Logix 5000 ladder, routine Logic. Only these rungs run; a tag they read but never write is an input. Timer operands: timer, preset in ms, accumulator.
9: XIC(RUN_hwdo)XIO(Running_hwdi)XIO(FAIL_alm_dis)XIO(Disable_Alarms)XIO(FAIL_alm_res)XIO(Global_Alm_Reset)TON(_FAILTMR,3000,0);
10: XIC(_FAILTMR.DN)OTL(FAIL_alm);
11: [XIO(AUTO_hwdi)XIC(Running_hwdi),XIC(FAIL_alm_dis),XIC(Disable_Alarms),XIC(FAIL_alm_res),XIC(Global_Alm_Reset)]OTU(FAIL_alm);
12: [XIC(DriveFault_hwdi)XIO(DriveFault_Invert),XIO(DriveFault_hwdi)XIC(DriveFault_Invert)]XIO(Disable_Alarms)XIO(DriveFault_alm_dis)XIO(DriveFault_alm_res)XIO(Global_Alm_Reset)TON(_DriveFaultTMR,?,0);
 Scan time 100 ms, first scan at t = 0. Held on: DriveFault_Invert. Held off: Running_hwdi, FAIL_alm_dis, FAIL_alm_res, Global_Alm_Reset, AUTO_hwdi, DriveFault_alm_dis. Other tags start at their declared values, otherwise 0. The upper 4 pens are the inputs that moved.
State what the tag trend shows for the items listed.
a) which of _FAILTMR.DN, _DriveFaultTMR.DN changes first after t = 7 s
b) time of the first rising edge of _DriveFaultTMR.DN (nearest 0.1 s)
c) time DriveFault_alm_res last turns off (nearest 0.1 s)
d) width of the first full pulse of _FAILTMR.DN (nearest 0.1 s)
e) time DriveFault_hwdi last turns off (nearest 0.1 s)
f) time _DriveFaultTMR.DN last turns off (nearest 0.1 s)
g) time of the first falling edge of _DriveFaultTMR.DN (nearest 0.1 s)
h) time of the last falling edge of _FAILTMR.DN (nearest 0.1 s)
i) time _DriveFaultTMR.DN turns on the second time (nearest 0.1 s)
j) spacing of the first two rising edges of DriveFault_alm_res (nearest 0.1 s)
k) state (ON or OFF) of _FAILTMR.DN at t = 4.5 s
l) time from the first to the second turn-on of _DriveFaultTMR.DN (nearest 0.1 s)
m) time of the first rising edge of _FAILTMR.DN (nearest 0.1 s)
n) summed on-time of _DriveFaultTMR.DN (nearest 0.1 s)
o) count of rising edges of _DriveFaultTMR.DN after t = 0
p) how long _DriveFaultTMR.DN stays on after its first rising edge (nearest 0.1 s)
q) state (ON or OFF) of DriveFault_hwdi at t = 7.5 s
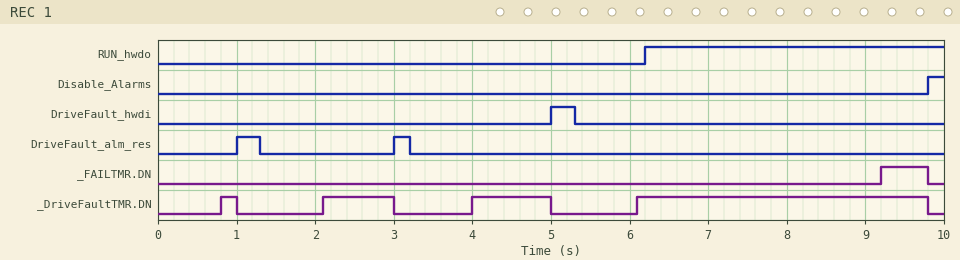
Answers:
_FAILTMR.DN
0.8 s
3.2 s
0.6 s
5.3 s
9.8 s
1.0 s
9.8 s
2.1 s
2.0 s
OFF
1.3 s
9.2 s
5.8 s
4
0.2 s
OFF
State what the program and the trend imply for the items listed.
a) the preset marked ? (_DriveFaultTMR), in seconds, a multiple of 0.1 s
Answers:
0.8 s
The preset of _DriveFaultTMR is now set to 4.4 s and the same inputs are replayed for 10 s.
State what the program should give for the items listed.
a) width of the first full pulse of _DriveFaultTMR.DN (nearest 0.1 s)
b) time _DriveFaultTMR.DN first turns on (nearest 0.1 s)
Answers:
0.1 s
9.7 s
